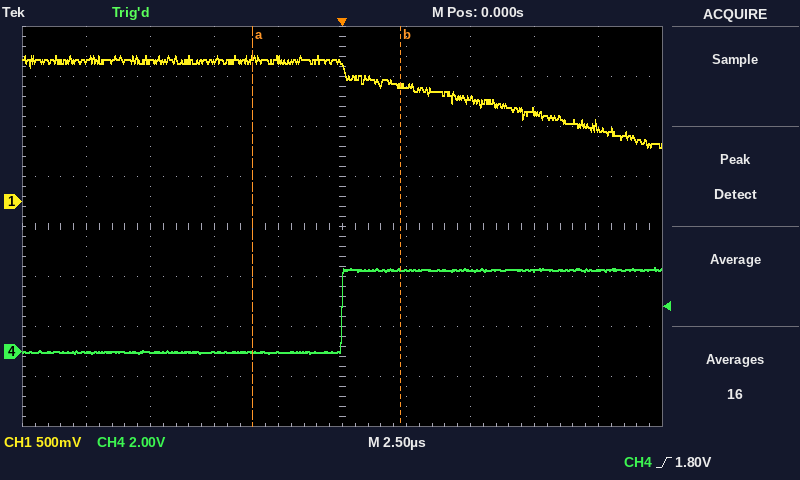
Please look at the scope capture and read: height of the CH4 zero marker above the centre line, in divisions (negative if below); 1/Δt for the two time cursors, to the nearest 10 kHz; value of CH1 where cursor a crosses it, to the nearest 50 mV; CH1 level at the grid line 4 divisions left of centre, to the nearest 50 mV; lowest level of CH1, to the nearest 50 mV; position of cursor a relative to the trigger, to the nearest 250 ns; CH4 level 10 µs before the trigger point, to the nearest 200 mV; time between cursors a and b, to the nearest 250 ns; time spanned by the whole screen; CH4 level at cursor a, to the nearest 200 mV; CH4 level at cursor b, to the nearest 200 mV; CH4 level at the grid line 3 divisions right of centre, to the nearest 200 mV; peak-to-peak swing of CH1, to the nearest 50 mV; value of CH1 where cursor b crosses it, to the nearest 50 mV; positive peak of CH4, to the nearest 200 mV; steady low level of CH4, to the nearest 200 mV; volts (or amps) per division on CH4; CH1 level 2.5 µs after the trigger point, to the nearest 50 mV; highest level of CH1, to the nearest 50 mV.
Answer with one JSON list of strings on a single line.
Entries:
["-2.5 div", "170 kHz", "1.40 V", "1.40 V", "550 mV", "-3.50 µs", "0.0 V", "5.75 µs", "25 µs", "0.0 V", "3.2 V", "3.2 V", "900 mV", "1.15 V", "3.4 V", "0.0 V", "2 V", "1.15 V", "1.45 V"]
